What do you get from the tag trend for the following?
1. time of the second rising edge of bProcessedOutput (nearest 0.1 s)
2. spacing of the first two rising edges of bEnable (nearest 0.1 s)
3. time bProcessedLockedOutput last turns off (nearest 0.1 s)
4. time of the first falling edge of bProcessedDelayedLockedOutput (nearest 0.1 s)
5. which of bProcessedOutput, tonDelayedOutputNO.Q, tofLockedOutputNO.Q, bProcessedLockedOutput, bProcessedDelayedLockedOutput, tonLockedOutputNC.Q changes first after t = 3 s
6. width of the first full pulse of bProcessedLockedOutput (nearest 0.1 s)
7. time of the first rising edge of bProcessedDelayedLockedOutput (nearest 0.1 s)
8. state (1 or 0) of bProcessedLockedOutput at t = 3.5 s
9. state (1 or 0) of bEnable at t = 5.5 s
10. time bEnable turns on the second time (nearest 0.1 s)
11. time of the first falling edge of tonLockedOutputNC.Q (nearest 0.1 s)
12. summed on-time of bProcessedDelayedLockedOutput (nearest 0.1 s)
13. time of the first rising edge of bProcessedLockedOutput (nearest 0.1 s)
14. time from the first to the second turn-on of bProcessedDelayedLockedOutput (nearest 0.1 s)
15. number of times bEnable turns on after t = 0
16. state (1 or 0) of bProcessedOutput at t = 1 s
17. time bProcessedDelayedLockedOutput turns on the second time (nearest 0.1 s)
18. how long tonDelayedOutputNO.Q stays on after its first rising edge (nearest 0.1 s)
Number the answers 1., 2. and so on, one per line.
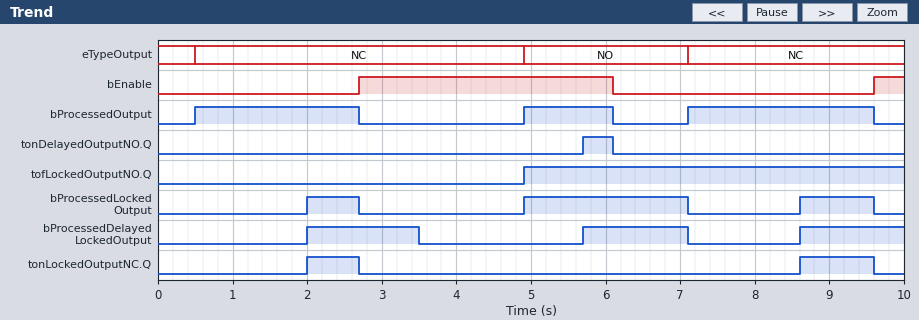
1. 4.9 s
2. 6.9 s
3. 9.6 s
4. 3.5 s
5. bProcessedDelayedLockedOutput
6. 0.7 s
7. 2.0 s
8. 0
9. 1
10. 9.6 s
11. 2.7 s
12. 4.3 s
13. 2.0 s
14. 3.7 s
15. 2
16. 1
17. 5.7 s
18. 0.4 s
